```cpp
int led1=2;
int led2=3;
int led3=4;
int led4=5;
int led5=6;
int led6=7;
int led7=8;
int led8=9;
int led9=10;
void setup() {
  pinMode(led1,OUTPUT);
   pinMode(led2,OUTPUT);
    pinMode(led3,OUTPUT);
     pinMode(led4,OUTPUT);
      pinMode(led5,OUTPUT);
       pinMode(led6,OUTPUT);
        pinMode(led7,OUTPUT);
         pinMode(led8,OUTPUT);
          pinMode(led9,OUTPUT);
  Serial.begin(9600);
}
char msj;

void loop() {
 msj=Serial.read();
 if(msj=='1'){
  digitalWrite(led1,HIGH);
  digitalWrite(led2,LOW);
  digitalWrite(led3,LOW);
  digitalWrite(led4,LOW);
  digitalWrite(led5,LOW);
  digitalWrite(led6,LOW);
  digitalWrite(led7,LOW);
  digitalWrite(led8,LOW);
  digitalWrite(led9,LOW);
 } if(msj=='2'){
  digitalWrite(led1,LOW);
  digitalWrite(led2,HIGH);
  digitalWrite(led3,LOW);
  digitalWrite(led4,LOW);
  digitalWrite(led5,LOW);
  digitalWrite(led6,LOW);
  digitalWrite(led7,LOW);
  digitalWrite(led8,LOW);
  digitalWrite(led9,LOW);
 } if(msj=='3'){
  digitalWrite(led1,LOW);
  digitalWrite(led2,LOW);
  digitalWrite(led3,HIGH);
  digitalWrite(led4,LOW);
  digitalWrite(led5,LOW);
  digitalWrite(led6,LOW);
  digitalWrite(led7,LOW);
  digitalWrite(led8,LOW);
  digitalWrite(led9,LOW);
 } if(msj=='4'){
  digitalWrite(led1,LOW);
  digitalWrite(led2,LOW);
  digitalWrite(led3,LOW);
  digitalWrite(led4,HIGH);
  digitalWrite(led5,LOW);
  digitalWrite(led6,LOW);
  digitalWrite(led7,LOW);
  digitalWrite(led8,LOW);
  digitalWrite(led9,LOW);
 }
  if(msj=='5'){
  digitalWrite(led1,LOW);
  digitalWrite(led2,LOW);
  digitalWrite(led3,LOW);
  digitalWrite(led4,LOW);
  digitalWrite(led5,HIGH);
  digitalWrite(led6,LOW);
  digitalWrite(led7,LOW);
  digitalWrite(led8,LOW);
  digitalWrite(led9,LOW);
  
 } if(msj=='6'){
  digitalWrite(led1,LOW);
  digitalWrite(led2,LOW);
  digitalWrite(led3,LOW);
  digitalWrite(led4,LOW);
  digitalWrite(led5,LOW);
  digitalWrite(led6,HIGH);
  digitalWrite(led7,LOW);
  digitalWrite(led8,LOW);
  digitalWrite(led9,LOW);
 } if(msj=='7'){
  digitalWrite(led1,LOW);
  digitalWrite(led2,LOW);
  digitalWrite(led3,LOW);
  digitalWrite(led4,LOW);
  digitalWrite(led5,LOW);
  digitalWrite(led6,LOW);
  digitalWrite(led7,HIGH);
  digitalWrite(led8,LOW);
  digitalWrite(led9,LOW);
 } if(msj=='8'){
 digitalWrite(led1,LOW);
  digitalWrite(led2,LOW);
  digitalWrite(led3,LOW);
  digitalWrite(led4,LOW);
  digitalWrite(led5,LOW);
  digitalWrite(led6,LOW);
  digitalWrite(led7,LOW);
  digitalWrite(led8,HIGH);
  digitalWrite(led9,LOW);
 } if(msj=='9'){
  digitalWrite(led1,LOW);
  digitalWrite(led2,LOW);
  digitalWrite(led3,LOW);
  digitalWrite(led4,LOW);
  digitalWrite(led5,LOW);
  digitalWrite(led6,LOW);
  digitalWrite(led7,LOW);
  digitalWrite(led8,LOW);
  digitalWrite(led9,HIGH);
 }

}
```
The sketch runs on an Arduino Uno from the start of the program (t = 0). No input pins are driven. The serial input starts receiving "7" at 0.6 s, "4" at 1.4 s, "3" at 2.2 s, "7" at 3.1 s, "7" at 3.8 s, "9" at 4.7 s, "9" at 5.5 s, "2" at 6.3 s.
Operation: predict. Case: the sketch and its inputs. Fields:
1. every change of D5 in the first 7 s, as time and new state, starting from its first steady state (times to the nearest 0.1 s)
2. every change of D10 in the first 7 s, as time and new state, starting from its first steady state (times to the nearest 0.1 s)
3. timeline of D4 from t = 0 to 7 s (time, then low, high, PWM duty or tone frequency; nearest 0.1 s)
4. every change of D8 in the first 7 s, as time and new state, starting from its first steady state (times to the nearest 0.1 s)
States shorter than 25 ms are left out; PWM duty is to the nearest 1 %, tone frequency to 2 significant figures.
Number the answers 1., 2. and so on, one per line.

1. 0 s low; 1.4 s high; 2.2 s low
2. 0 s low; 4.7 s high; 6.3 s low
3. 0 s low; 2.2 s high; 3.1 s low
4. 0 s low; 0.6 s high; 1.4 s low; 3.1 s high; 4.7 s low
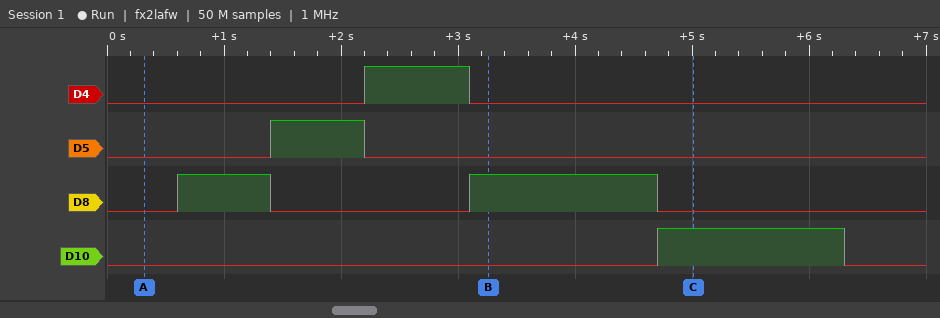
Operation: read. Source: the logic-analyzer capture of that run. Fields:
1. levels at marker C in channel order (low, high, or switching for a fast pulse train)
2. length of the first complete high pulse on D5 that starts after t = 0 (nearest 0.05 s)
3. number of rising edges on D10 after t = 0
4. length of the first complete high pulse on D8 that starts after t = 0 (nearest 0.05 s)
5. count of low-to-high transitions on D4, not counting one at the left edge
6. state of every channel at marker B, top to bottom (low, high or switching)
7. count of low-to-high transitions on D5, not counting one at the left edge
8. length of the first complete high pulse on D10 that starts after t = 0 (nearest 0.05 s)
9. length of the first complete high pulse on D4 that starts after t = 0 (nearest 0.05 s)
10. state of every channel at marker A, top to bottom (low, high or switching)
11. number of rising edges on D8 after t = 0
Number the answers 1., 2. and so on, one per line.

1. D4 low, D5 low, D8 low, D10 high
2. 0.80 s
3. 1
4. 0.80 s
5. 1
6. D4 low, D5 low, D8 high, D10 low
7. 1
8. 1.60 s
9. 0.90 s
10. D4 low, D5 low, D8 low, D10 low
11. 2
